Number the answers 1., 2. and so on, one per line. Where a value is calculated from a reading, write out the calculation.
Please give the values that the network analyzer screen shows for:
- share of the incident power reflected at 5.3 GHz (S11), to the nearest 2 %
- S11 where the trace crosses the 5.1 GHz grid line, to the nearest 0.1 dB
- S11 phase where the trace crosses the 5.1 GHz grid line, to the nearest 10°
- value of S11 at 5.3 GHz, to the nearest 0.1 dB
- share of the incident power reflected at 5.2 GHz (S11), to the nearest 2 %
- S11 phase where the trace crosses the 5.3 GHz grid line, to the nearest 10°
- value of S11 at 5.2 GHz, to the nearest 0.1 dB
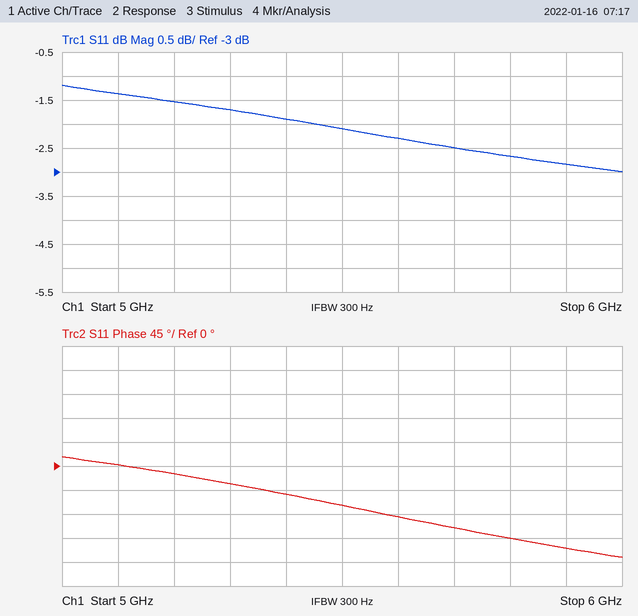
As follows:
1. 10^(-1.7/10) ≈ 68 %
2. -1.4 dB
3. 0°
4. -1.7 dB
5. 10^(-1.5/10) ≈ 70.8 %, so 70 % to the nearest 2 %
6. -30°
7. -1.5 dB
